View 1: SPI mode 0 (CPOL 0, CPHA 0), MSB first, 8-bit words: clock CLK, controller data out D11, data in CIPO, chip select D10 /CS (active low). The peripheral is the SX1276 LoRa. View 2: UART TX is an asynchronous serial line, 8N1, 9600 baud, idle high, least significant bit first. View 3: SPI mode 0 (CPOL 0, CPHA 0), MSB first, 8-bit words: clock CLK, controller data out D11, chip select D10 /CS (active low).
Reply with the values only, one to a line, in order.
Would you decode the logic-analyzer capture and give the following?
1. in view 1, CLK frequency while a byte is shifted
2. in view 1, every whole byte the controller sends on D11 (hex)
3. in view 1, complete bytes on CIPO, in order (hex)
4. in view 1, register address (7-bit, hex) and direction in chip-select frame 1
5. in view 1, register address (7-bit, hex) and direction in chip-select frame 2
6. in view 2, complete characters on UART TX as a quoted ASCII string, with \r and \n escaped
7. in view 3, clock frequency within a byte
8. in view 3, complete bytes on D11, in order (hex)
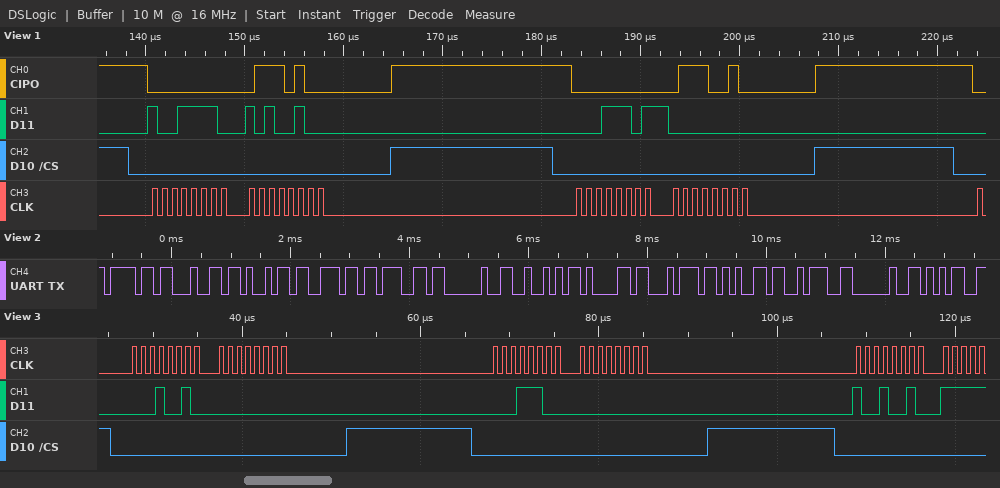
1 MHz
9E A4 1D 00
00 74 00 72
0x1E write
0x1D read
"oding Rate: 5"
1 MHz
0x12 0x00 0x1C 0x00 0x92
